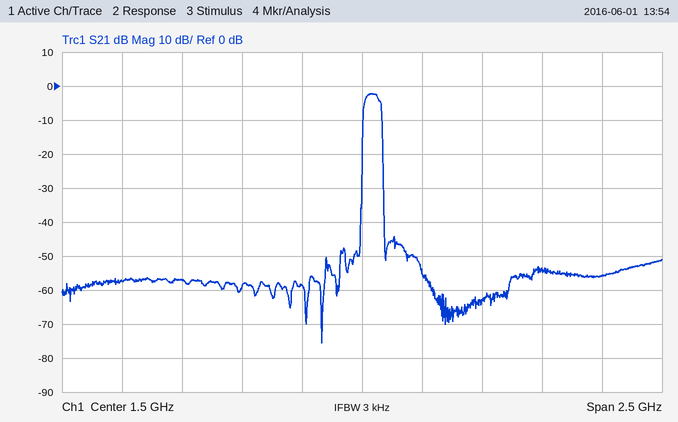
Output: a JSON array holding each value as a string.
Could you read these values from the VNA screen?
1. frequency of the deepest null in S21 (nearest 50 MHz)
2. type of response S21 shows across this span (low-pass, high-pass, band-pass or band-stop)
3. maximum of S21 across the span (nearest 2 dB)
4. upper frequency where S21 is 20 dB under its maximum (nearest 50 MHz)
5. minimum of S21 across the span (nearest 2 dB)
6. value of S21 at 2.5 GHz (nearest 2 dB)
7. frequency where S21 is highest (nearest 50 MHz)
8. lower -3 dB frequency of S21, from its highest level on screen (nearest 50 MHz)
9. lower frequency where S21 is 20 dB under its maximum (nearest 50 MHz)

["1.35 GHz", "band-pass", "-2 dB", "1.60 GHz", "-76 dB", "-56 dB", "1.55 GHz", "1.50 GHz", "1.50 GHz"]
